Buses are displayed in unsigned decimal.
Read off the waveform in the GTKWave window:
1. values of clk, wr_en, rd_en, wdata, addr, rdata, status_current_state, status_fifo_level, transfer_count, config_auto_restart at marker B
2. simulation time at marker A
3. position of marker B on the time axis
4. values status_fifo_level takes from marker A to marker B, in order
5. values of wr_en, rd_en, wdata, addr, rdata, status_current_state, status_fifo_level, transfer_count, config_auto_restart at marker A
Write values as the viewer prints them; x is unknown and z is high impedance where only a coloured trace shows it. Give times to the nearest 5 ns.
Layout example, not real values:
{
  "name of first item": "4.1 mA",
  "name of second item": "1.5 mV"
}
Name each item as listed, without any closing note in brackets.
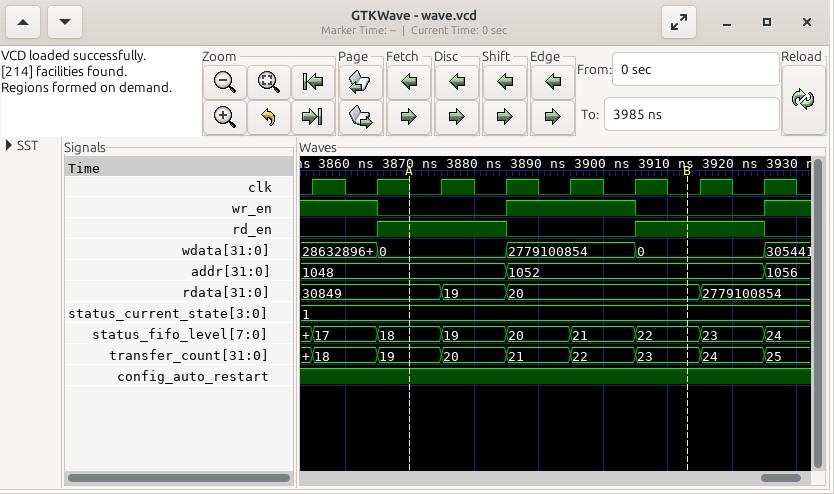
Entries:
{
  "values of clk, wr_en, rd_en, wdata, addr, rdata, status_current_state, status_fifo_level, transfer_count, config_auto_restart at marker B": "clk=0, wr_en=0, rd_en=1, wdata=0, addr=1052, rdata=20, status_current_state=1, status_fifo_level=22, transfer_count=23, config_auto_restart=1",
  "simulation time at marker A": "3870 ns",
  "position of marker B on the time axis": "3915 ns",
  "values status_fifo_level takes from marker A to marker B, in order": "18, 19, 20, 21, 22",
  "values of wr_en, rd_en, wdata, addr, rdata, status_current_state, status_fifo_level, transfer_count, config_auto_restart at marker A": "wr_en=0, rd_en=1, wdata=0, addr=1048, rdata=30849, status_current_state=1, status_fifo_level=18, transfer_count=19, config_auto_restart=1"
}
